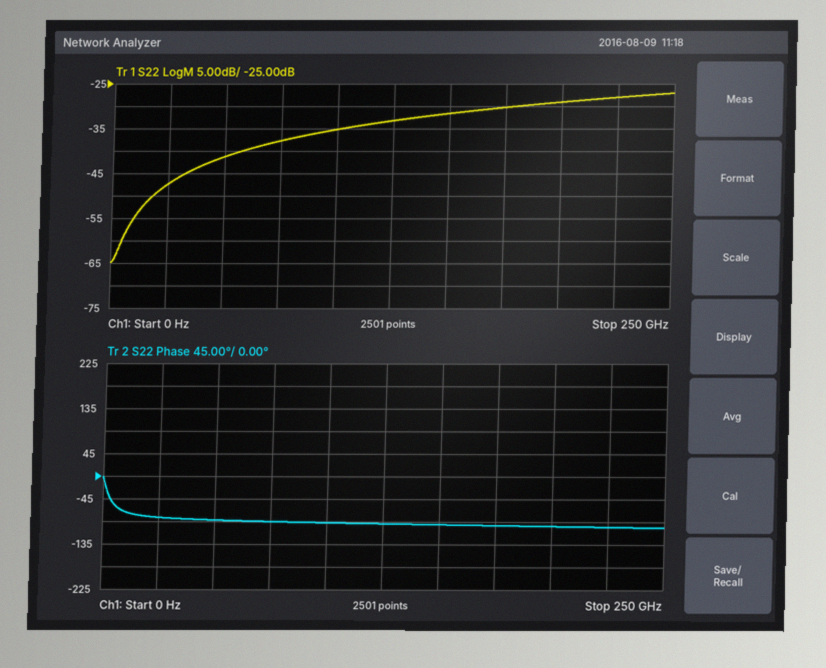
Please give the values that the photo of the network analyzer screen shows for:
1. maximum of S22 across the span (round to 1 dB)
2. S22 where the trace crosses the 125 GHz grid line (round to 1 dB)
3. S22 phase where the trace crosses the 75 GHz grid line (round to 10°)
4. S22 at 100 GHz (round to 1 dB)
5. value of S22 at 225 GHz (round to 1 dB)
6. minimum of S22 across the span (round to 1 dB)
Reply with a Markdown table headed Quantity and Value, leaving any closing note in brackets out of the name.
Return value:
| Quantity | Value |
|---|---|
| maximum of S22 across the span | -27 dB |
| S22 where the trace crosses the 125 GHz grid line | -33 dB |
| S22 phase where the trace crosses the 75 GHz grid line | -90° |
| S22 at 100 GHz | -35 dB |
| value of S22 at 225 GHz | -28 dB |
| minimum of S22 across the span | -65 dB |
